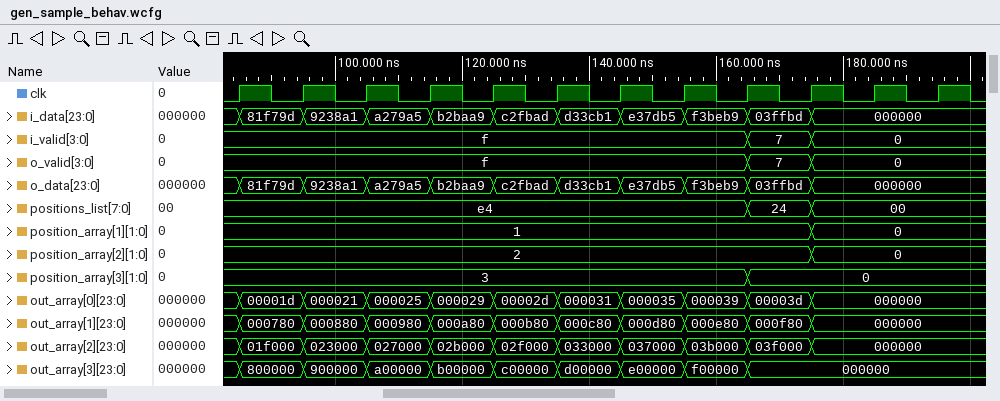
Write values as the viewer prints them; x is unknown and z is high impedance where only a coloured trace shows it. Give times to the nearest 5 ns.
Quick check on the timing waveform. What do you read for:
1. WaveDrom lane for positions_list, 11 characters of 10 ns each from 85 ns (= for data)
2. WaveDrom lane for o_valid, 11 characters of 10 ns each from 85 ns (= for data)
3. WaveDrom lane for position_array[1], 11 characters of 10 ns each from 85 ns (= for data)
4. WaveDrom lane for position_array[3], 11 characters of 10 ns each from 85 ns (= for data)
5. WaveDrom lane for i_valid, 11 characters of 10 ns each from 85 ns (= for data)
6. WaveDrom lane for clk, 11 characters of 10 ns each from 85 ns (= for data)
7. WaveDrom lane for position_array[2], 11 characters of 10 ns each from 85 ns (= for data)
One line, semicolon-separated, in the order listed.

{name: 'positions_list', wave: '=.......==.', data: 'e4 24 00'}; {name: 'o_valid', wave: '=.......==.', data: 'f 7 0'}; {name: 'position_array[1]', wave: '=........=.', data: '1 0'}; {name: 'position_array[3]', wave: '=.......=..', data: '3 0'}; {name: 'i_valid', wave: '=.......==.', data: 'f 7 0'}; {name: 'clk', wave: 'p..........'}; {name: 'position_array[2]', wave: '=........=.', data: '2 0'}
